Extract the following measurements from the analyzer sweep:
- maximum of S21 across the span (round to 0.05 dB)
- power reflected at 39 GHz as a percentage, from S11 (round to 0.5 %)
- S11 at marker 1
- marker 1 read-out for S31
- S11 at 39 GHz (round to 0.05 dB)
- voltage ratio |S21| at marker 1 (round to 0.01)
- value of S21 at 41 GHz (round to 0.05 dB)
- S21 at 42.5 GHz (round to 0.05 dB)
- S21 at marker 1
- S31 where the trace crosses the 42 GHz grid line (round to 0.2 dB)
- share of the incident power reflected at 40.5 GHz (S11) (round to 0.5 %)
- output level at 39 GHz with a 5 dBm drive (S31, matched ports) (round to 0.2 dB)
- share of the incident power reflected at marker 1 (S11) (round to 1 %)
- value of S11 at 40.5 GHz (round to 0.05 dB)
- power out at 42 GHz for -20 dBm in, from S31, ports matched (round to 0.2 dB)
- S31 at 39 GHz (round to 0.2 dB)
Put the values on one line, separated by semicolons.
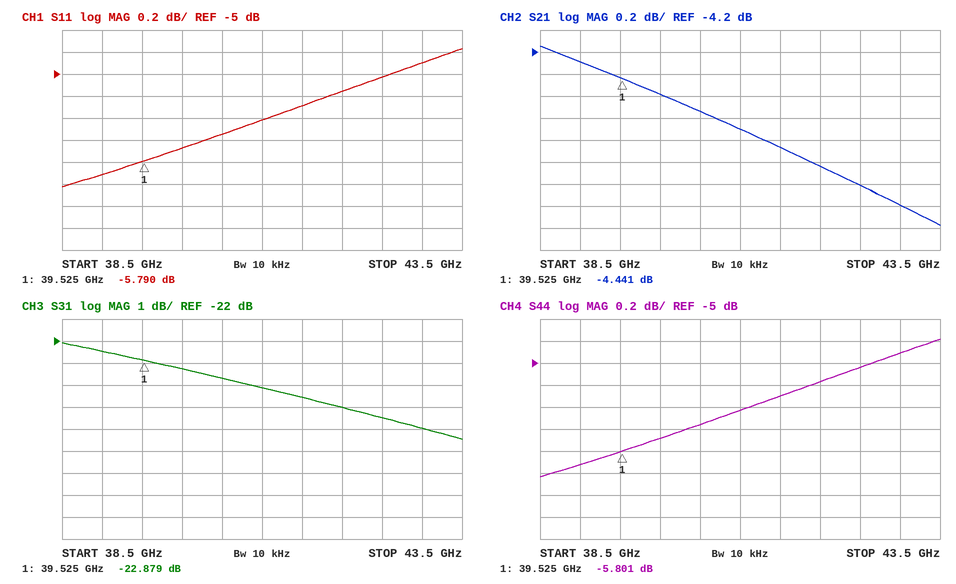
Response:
-4.15 dB; 25.5 %; -5.790 dB; -22.879 dB; -5.90 dB; 0.60; -4.90 dB; -5.40 dB; -4.441 dB; -25.0 dB; 28.0 %; -17.4 dBm; 26 %; -5.55 dB; -45.0 dBm; -22.4 dB
